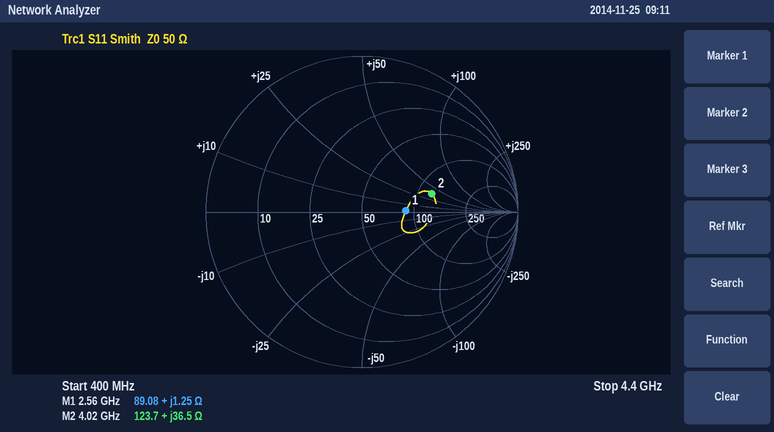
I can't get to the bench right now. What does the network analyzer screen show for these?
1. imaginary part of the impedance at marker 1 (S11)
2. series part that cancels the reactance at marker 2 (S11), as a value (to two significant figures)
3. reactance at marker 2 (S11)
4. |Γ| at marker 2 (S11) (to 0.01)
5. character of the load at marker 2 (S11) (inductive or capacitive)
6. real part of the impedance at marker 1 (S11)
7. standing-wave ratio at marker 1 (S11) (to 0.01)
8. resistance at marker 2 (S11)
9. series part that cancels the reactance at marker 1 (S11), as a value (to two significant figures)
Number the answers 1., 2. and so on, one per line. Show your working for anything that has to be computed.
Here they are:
1. +1.25 Ω
2. C = 1/(2π × 4.02 GHz × 36.5 Ω) ≈ 1.1 pF
3. +36.5 Ω
4. 0.46
5. inductive
6. 89.08 Ω
7. 1.78
8. 123.7 Ω
9. C = 1/(2π × 2.56 GHz × 1.25 Ω) ≈ 50 pF
